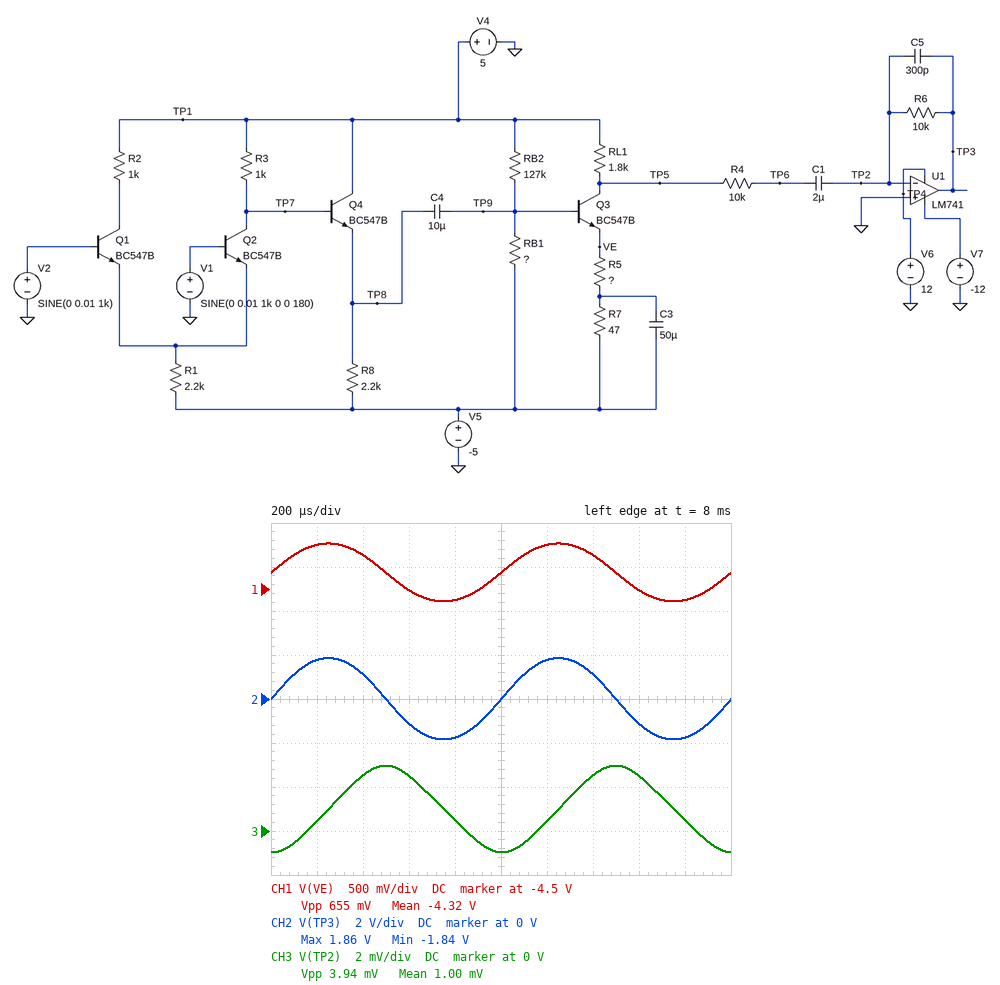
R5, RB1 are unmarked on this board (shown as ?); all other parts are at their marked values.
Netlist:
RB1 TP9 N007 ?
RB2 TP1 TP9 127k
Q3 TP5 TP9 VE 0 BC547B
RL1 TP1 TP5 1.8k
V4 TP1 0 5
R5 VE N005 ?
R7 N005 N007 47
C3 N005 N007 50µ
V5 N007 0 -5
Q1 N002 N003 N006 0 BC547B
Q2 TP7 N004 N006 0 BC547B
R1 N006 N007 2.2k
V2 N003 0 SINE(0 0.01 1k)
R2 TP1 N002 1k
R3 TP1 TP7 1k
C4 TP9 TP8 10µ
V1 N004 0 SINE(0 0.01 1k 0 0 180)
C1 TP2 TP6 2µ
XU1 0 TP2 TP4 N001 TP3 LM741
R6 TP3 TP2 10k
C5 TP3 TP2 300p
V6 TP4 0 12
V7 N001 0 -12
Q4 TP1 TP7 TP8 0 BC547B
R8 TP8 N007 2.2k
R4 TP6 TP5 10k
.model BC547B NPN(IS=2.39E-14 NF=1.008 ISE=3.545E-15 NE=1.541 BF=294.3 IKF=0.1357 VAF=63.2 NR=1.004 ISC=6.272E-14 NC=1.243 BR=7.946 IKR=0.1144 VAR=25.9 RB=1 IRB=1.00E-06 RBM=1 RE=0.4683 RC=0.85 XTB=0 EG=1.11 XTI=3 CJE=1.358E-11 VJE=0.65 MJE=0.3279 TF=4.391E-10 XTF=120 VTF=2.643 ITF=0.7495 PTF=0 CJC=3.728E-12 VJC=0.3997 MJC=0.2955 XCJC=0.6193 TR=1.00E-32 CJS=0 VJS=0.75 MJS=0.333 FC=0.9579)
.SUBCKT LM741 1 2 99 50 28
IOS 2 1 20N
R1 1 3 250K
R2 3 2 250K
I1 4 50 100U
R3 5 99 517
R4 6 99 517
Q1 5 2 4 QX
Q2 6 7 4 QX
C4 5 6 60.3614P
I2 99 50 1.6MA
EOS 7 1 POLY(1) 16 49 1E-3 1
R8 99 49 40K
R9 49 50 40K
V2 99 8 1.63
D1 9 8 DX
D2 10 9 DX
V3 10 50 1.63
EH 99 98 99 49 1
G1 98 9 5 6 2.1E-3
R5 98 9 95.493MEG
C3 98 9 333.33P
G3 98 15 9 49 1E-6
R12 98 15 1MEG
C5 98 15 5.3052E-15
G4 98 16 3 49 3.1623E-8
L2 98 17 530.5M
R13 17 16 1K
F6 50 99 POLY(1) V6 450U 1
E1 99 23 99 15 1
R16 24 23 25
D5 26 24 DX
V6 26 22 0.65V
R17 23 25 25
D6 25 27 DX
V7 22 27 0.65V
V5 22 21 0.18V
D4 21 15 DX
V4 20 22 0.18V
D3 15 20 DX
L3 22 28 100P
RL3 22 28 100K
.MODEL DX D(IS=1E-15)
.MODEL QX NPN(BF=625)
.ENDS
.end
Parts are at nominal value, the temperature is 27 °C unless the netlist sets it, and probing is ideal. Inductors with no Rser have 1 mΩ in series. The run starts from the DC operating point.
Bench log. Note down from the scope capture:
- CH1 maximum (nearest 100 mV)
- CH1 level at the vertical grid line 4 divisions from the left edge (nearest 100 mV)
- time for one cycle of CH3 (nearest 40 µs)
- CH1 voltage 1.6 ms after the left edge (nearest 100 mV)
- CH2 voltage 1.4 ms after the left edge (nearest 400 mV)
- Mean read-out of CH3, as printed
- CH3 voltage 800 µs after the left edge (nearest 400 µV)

-4.0 V
-4.6 V
1.00 ms
-4.5 V
1.2 V
1.00 mV
400 µV
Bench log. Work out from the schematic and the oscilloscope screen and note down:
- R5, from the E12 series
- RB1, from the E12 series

270 Ω
22 kΩ
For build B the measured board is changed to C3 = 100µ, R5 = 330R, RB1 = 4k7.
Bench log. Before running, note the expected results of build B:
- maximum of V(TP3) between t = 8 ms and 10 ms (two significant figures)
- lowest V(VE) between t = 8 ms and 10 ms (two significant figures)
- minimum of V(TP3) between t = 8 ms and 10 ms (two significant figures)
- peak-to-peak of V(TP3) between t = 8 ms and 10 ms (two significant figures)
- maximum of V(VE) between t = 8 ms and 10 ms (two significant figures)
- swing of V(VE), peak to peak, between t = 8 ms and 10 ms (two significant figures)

420 mV
-5.0 V
-30 mV
450 mV
-4.9 V
97 mV
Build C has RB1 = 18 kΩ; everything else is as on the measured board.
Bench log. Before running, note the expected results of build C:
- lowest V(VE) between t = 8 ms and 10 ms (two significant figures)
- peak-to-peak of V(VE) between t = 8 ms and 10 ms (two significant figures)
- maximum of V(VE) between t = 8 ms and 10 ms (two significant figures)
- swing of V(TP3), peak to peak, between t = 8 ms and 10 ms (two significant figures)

-4.8 V
640 mV
-4.2 V
3.6 V
